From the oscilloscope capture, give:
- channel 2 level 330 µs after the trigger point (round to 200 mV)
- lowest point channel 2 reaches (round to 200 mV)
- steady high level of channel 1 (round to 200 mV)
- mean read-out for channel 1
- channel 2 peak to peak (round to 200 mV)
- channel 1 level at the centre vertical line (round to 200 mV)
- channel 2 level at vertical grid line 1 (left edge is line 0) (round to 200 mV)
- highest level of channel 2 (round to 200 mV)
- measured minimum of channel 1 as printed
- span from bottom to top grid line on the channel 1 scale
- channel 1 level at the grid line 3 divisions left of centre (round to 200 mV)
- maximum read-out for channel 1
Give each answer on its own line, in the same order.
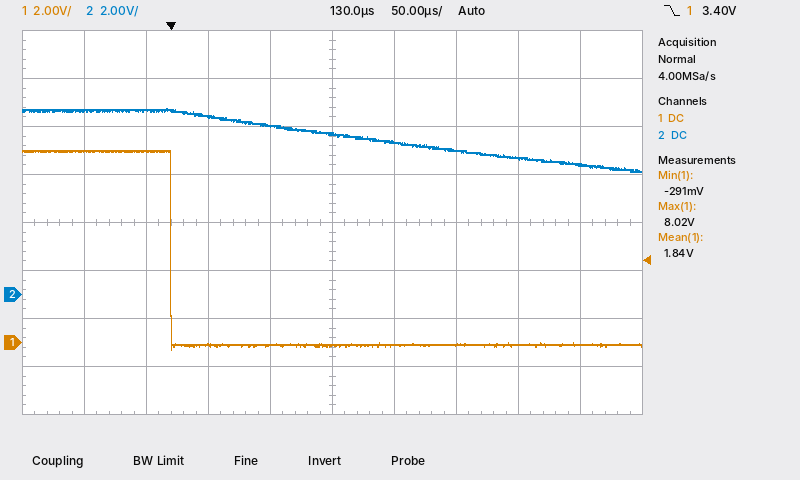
5.4 V
5.2 V
8.0 V
1.84 V
2.6 V
-200 mV
7.6 V
7.8 V
-291 mV
16 V
8.0 V
8.02 V
